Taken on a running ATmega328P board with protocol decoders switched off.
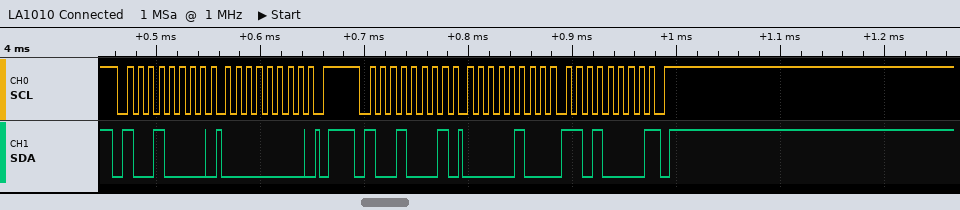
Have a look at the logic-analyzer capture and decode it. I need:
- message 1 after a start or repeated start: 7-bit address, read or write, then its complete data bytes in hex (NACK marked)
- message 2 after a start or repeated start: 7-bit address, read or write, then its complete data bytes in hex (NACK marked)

0x48 write: 00
0x48 read: 04 D0 NACK
